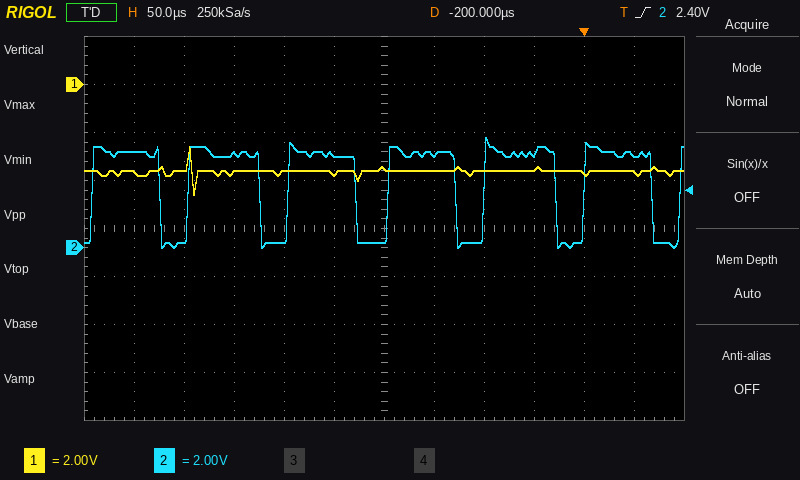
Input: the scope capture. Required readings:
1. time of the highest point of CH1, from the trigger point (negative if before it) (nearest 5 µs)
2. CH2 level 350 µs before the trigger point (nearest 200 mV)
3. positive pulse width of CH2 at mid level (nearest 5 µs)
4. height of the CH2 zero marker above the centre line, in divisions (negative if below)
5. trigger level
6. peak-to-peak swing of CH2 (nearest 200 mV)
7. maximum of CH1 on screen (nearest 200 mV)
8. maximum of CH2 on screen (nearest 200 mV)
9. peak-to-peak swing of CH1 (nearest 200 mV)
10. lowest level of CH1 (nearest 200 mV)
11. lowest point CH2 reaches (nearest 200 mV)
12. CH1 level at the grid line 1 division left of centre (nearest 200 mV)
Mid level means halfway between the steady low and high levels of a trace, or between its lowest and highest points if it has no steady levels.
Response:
-395 µs
4.0 V
70 µs
-0.4 div
2.40 V
4.6 V
-2.6 V
4.6 V
2.0 V
-4.6 V
0.0 V
-3.8 V
